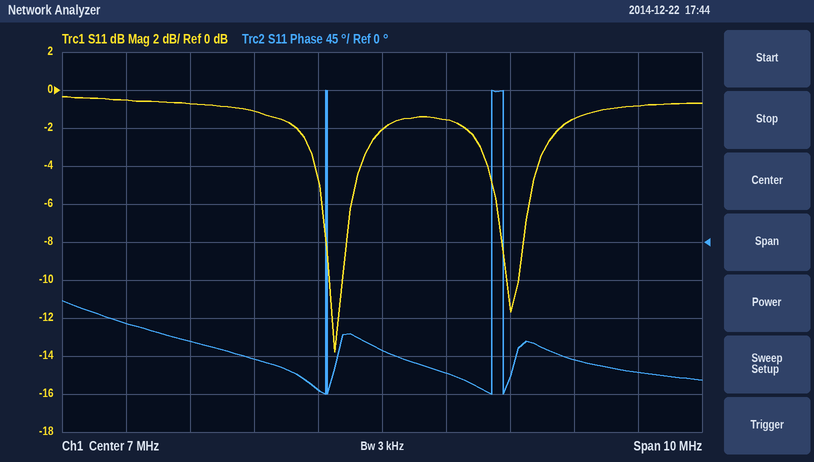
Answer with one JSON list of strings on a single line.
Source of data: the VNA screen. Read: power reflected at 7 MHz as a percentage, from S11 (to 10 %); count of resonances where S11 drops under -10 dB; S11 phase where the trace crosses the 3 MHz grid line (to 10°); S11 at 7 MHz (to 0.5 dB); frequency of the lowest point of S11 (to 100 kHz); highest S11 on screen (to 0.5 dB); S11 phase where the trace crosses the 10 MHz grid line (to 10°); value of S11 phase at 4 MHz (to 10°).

["60 %", "2", "-100°", "-2.0 dB", "6.3 MHz", "-0.5 dB", "-140°", "-120°"]
